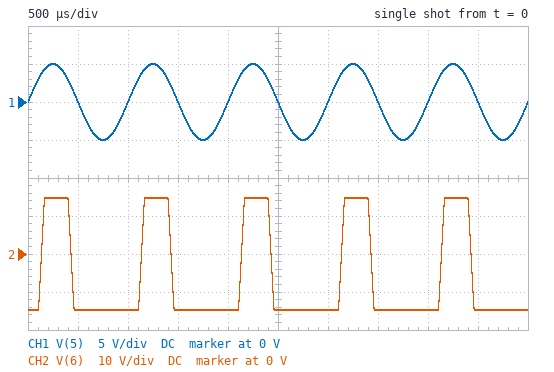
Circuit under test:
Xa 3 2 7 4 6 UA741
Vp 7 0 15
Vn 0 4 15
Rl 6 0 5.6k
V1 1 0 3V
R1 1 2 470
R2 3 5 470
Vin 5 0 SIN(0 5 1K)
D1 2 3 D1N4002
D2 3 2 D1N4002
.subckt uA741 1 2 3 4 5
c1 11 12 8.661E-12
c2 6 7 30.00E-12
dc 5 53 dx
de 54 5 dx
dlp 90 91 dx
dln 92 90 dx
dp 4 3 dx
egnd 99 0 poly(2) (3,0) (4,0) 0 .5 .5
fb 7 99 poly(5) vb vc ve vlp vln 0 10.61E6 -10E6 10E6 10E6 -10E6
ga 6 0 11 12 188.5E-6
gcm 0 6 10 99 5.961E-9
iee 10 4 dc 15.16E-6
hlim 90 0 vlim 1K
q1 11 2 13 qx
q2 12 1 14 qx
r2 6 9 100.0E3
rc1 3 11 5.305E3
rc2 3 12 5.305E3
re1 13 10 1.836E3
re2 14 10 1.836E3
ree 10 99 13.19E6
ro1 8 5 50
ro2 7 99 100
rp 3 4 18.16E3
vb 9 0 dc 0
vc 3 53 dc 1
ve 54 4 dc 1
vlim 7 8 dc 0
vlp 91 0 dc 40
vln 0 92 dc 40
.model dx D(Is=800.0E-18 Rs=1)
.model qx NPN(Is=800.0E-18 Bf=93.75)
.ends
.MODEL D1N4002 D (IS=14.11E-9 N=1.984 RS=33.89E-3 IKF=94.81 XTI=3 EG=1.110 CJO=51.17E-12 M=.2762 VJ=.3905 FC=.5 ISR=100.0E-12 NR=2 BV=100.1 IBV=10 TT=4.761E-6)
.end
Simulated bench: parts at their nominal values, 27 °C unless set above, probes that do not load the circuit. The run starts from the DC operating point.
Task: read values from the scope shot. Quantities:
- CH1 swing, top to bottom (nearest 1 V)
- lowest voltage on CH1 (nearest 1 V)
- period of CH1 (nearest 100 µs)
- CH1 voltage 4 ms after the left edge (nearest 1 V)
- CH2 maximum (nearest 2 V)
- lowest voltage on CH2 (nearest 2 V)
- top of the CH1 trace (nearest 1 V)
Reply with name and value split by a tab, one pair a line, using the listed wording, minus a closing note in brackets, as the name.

CH1 swing, top to bottom	10 V
lowest voltage on CH1	-5 V
period of CH1	1.0 ms
CH1 voltage 4 ms after the left edge	0 V
CH2 maximum	14 V
lowest voltage on CH2	-14 V
top of the CH1 trace	5 V
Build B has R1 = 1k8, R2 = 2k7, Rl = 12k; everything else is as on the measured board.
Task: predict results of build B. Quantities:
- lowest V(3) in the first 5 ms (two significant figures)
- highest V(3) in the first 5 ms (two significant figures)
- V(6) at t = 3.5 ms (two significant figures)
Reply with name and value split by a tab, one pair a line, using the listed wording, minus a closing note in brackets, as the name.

lowest V(3) in the first 5 ms	-560 mV
highest V(3) in the first 5 ms	4.1 V
V(6) at t = 3.5 ms	-15 V
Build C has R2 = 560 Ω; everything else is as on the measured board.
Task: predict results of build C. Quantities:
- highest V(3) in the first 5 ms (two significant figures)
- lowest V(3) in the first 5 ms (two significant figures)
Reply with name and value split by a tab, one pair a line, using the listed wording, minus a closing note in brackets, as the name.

highest V(3) in the first 5 ms	4.2 V
lowest V(3) in the first 5 ms	-1.0 V
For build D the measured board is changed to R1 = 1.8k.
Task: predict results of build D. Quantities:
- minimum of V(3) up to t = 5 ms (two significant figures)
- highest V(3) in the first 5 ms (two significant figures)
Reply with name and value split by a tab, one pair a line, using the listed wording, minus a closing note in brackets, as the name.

minimum of V(3) up to t = 5 ms	-3.5 V
highest V(3) in the first 5 ms	4.7 V
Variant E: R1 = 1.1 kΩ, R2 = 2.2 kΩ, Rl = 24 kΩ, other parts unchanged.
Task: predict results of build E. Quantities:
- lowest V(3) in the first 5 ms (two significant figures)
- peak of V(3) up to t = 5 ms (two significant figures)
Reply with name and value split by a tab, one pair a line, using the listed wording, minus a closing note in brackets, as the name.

lowest V(3) in the first 5 ms	-76 mV
peak of V(3) up to t = 5 ms	4.0 V
